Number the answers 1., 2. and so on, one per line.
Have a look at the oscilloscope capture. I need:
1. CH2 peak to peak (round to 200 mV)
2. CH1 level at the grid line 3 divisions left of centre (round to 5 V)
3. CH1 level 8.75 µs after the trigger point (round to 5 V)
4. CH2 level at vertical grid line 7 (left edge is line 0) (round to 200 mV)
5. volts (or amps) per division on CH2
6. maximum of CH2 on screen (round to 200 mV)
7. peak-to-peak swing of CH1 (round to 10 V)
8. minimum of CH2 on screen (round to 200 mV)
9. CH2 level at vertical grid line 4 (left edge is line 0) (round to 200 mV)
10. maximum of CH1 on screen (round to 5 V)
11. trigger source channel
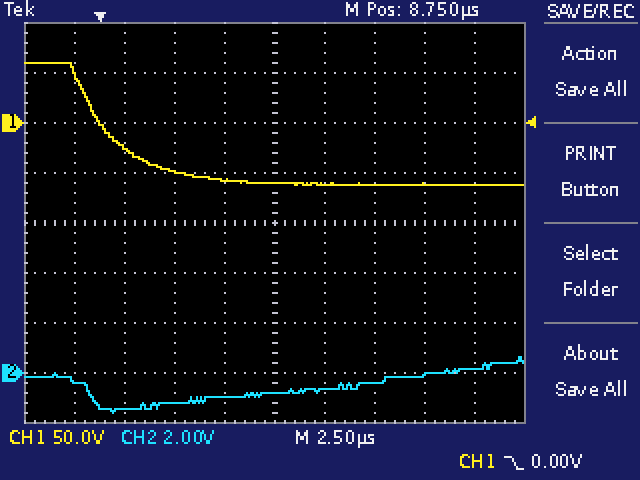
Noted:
1. 2.2 V
2. -25 V
3. -60 V
4. -400 mV
5. 2 V
6. 600 mV
7. 120 V
8. -1.6 V
9. -1.0 V
10. 60 V
11. CH1
